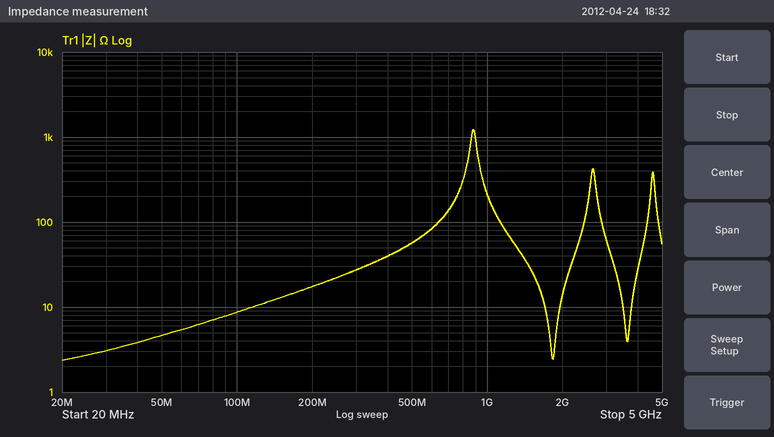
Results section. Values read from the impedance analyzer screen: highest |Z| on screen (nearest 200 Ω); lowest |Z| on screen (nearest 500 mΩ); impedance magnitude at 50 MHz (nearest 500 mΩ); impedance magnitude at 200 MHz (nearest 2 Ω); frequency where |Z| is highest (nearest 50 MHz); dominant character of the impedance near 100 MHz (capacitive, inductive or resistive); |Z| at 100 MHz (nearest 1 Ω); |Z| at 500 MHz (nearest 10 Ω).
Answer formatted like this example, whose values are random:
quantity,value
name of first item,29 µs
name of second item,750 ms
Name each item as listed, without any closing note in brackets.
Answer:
quantity,value
highest |Z| on screen,1.2 kΩ
lowest |Z| on screen,2.5 Ω
impedance magnitude at 50 MHz,4.5 Ω
impedance magnitude at 200 MHz,18 Ω
frequency where |Z| is highest,900 MHz
dominant character of the impedance near 100 MHz,inductive
|Z| at 100 MHz,9 Ω
|Z| at 500 MHz,60 Ω
